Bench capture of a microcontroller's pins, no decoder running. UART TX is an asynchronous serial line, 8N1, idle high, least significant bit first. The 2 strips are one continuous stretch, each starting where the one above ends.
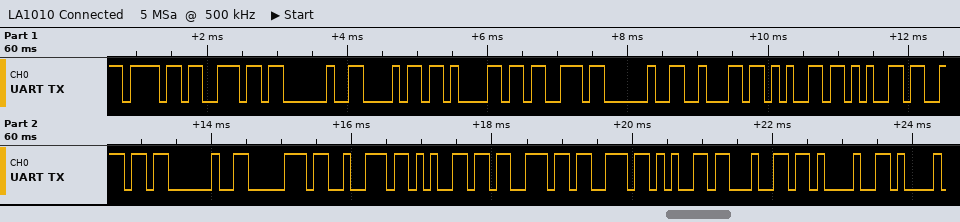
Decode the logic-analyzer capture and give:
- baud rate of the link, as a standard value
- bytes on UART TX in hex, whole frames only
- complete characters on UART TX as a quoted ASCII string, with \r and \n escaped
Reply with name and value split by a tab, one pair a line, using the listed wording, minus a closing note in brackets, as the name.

baud rate of the link, as a standard value	9600 baud
bytes on UART TX in hex, whole frames only	0x6F 0x6E 0x20 0x68 0x61 0x73 0x20 0x62 0x65 0x65 0x6E 0x20 0x70 0x72 0x65 0x73 0x73 0x65 0x64 0x21
complete characters on UART TX as a quoted ASCII string, with \r and \n escaped	"on has been pressed!"
